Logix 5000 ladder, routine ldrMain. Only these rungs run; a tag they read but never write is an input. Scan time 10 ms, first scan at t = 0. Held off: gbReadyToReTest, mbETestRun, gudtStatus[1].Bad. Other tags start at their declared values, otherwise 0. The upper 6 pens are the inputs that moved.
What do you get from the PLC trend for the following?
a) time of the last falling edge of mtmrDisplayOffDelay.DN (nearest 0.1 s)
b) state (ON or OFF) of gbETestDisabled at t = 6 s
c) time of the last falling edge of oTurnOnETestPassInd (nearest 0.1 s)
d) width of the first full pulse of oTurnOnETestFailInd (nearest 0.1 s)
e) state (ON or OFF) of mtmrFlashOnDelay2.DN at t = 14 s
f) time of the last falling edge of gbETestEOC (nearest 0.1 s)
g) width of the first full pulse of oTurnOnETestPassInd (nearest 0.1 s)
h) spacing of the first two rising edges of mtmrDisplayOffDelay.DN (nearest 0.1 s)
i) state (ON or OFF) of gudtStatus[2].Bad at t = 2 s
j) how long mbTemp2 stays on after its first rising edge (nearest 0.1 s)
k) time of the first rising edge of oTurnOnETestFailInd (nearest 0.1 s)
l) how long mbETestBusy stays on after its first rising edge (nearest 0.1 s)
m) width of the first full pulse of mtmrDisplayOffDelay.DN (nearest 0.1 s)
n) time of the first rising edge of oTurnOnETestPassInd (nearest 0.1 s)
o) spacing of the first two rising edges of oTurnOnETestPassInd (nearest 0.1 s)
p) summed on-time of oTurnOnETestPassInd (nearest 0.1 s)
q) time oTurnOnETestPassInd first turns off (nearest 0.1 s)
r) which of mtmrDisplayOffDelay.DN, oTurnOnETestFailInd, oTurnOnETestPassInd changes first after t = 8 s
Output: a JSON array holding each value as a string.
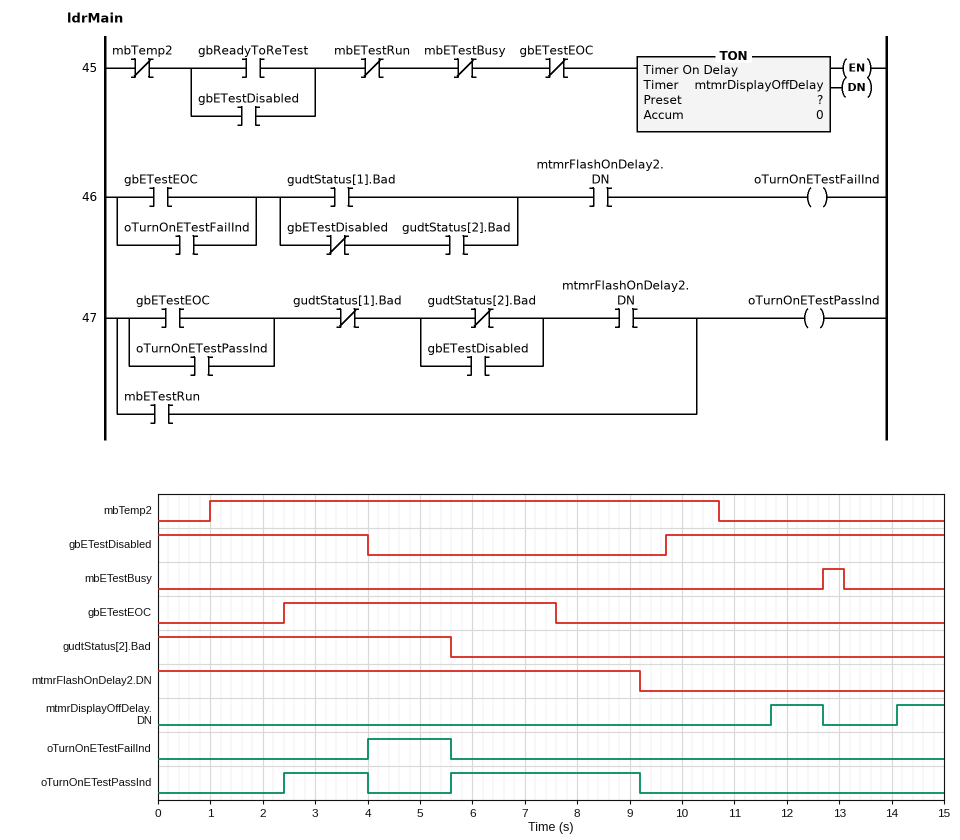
["12.7 s", "OFF", "9.2 s", "1.6 s", "OFF", "7.6 s", "1.6 s", "2.4 s", "ON", "9.7 s", "4.0 s", "0.4 s", "1.0 s", "2.4 s", "3.2 s", "5.2 s", "4.0 s", "oTurnOnETestPassInd"]
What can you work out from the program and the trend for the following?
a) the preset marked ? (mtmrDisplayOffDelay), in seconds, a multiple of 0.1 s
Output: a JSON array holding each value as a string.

["1.0 s"]
